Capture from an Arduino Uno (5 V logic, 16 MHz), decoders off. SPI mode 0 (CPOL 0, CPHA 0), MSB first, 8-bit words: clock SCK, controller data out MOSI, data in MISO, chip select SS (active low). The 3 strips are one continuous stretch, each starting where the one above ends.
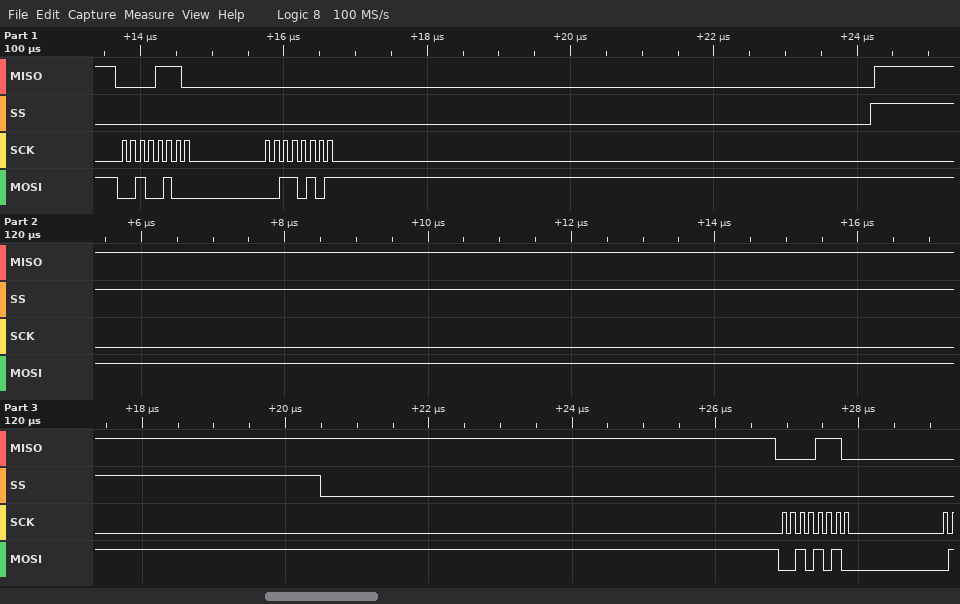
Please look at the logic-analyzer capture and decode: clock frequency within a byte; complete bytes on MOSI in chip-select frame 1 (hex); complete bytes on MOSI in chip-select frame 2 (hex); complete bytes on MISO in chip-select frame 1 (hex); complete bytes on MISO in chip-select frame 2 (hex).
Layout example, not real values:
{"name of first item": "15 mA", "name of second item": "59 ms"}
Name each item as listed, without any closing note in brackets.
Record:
{"clock frequency within a byte": "8 MHz", "complete bytes on MOSI in chip-select frame 1": "24 35", "complete bytes on MOSI in chip-select frame 2": "2A", "complete bytes on MISO in chip-select frame 1": "0E 00", "complete bytes on MISO in chip-select frame 2": "0E"}
